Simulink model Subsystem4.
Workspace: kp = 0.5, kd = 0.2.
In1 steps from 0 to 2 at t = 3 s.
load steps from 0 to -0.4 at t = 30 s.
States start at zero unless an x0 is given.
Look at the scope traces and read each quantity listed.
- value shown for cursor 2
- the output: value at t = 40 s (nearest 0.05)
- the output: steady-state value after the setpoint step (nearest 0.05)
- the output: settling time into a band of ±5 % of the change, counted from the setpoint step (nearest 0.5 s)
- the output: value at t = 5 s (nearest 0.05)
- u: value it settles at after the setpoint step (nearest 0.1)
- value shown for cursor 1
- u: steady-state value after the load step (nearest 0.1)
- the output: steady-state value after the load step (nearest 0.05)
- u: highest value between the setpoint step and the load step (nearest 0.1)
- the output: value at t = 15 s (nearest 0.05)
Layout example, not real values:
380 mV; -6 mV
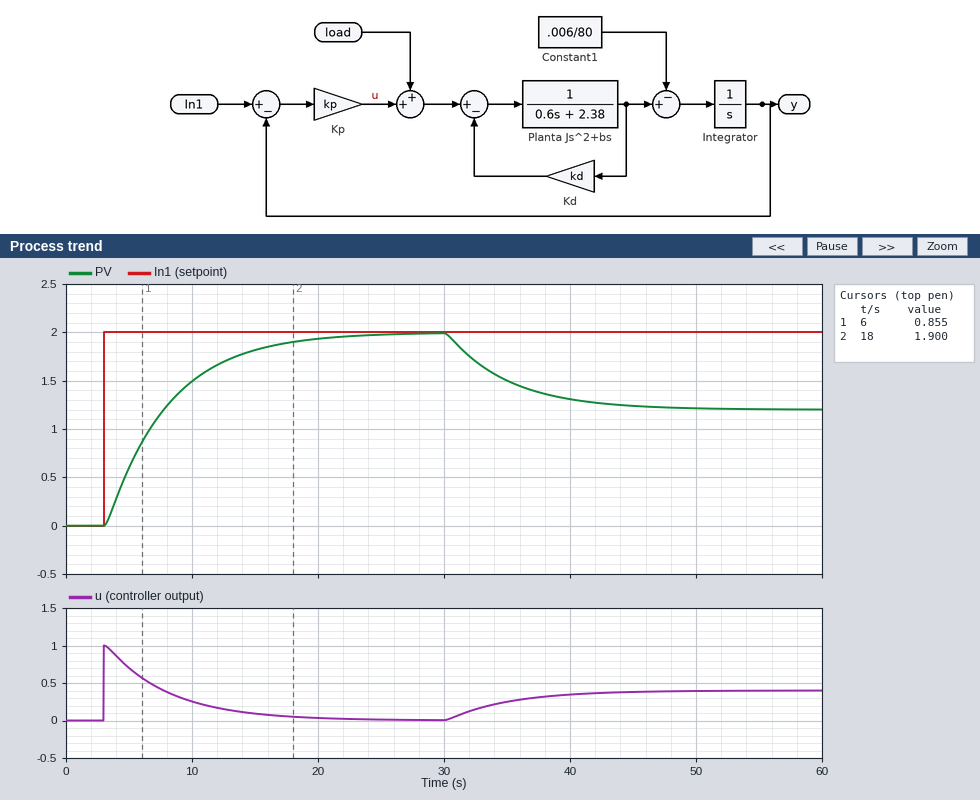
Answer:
1.900; 1.30; 2.00; 15.0 s; 0.60; 0.0; 0.855; 0.4; 1.20; 1.0; 1.80
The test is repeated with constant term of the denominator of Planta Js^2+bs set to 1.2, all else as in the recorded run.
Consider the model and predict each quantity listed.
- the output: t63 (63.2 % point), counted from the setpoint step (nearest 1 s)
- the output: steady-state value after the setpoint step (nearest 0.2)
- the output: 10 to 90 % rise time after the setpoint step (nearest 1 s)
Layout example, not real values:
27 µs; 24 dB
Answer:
3 s; 2.0; 5 s
